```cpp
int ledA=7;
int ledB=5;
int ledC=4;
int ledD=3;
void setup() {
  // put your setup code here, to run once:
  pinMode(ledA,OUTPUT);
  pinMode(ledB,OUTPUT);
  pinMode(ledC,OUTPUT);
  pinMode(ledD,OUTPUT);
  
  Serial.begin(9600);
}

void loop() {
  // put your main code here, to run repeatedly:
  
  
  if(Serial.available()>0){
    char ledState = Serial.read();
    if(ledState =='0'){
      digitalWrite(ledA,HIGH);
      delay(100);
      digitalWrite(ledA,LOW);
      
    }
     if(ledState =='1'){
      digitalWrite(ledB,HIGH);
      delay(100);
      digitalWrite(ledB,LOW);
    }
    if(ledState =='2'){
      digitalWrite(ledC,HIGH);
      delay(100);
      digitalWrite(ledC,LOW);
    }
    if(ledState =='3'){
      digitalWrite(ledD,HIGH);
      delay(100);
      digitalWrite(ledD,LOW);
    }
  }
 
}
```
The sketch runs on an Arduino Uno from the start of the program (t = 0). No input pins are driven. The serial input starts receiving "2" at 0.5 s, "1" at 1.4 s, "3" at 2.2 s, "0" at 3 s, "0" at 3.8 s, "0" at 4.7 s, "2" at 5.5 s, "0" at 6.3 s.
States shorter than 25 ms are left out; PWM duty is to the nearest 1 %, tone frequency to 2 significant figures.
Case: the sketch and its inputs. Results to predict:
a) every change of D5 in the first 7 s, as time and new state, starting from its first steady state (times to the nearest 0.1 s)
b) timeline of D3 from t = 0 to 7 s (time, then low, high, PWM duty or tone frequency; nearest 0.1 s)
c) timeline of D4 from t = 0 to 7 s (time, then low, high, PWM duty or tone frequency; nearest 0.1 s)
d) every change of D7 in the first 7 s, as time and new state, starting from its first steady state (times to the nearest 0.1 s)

0 s low; 1.4 s high; 1.5 s low
0 s low; 2.2 s high; 2.3 s low
0 s low; 0.5 s high; 0.6 s low; 5.5 s high; 5.6 s low
0 s low; 3 s high; 3.1 s low; 3.8 s high; 3.9 s low; 4.7 s high; 4.8 s low; 6.3 s high; 6.4 s low
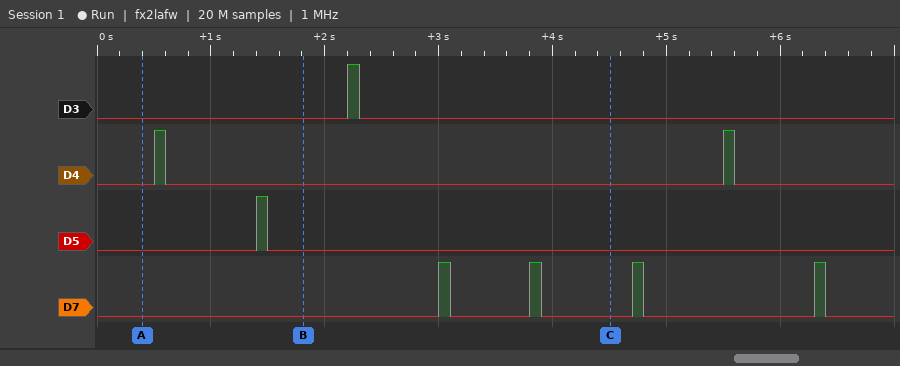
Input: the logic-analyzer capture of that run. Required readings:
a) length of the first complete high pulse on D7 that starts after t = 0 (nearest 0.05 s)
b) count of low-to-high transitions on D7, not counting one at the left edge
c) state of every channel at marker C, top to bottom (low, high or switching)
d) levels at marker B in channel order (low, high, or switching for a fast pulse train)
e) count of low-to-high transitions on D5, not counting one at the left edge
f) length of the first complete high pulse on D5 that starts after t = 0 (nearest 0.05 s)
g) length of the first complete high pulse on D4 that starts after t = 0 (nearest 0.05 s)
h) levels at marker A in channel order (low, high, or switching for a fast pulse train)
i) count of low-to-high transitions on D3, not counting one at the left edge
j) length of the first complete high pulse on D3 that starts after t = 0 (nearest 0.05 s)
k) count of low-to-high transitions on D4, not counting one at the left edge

0.10 s
4
D3 low, D4 low, D5 low, D7 low
D3 low, D4 low, D5 low, D7 low
1
0.10 s
0.10 s
D3 low, D4 low, D5 low, D7 low
1
0.10 s
2
